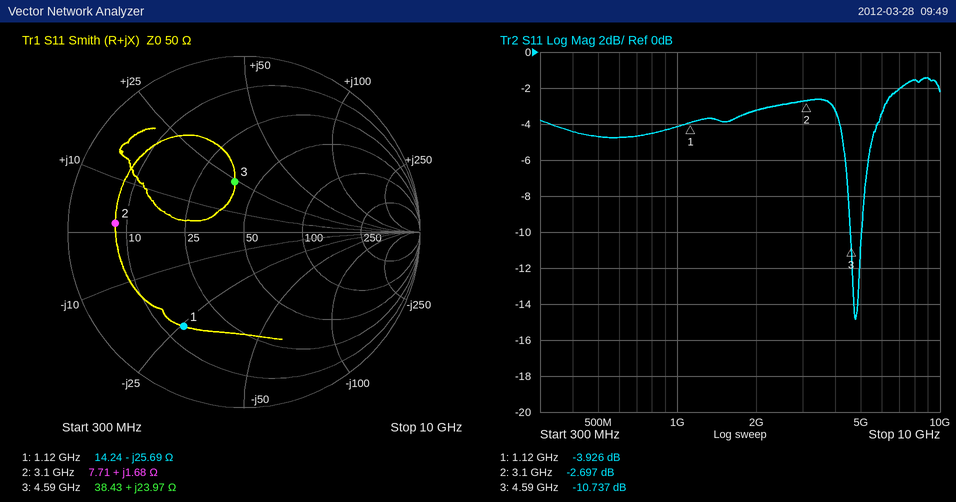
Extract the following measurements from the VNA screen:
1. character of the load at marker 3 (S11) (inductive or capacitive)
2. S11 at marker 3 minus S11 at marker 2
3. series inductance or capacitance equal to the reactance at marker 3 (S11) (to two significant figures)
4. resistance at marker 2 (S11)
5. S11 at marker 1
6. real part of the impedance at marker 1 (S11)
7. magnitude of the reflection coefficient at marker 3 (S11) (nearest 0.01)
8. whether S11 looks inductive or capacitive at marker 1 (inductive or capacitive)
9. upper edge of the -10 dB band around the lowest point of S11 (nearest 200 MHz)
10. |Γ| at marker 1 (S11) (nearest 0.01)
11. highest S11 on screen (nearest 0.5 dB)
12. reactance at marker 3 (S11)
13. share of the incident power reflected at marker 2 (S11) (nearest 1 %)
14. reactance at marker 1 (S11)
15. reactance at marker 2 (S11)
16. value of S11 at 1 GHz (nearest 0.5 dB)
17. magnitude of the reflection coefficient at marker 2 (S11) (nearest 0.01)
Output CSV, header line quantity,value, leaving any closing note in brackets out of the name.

quantity,value
character of the load at marker 3 (S11),inductive
S11 at marker 3 minus S11 at marker 2,-8.040 dB
series inductance or capacitance equal to the reactance at marker 3 (S11),830 pH
resistance at marker 2,7.71 Ω
S11 at marker 1,-3.926 dB
real part of the impedance at marker 1,14.24 Ω
magnitude of the reflection coefficient at marker 3 (S11),0.29
whether S11 looks inductive or capacitive at marker 1,capacitive
upper edge of the -10 dB band around the lowest point of S11,5.0 GHz
|Γ| at marker 1 (S11),0.64
highest S11 on screen,-1.5 dB
reactance at marker 3,+23.97 Ω
share of the incident power reflected at marker 2 (S11),54 %
reactance at marker 1,-25.69 Ω
reactance at marker 2,+1.68 Ω
value of S11 at 1 GHz,-4.0 dB
magnitude of the reflection coefficient at marker 2 (S11),0.73
